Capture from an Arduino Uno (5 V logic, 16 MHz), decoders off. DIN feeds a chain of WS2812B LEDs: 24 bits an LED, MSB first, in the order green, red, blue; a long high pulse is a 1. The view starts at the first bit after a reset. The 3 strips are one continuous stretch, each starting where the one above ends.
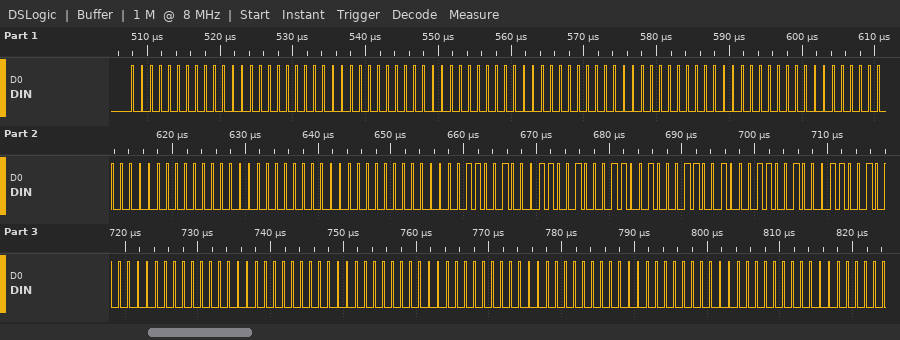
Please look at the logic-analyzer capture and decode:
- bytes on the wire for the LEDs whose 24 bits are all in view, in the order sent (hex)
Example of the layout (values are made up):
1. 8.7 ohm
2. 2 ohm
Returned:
1. 00 00 00 00 00 00 00 00 00 00 00 00 00 00 00 32 32 32 32 32 32 00 00 00 00 00 00 00 00 00
